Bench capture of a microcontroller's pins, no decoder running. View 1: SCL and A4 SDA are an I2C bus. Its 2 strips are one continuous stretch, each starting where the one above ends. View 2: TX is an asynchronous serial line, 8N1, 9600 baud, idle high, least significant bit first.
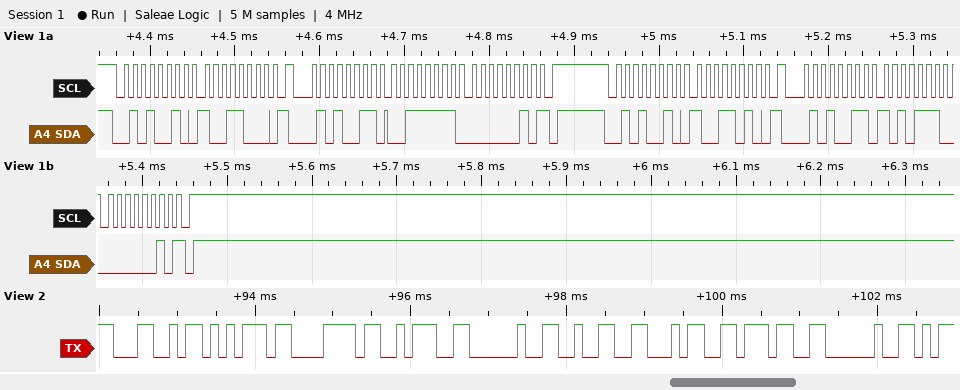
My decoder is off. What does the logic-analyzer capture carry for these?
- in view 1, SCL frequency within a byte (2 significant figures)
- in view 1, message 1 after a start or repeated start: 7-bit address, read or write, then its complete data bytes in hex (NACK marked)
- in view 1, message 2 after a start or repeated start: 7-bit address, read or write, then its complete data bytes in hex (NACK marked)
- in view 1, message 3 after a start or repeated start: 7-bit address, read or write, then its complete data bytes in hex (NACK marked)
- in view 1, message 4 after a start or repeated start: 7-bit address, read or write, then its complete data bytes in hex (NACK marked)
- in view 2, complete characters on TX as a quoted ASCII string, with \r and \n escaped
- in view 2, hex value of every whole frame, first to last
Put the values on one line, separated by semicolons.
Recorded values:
100 kHz; 0x29 write: 98; 0x29 read: 3F 02 NACK; 0x29 write: 9A; 0x29 read: AE 02 NACK; "Lux: 247 "; 4C 75 78 3A 20 32 34 37 20
